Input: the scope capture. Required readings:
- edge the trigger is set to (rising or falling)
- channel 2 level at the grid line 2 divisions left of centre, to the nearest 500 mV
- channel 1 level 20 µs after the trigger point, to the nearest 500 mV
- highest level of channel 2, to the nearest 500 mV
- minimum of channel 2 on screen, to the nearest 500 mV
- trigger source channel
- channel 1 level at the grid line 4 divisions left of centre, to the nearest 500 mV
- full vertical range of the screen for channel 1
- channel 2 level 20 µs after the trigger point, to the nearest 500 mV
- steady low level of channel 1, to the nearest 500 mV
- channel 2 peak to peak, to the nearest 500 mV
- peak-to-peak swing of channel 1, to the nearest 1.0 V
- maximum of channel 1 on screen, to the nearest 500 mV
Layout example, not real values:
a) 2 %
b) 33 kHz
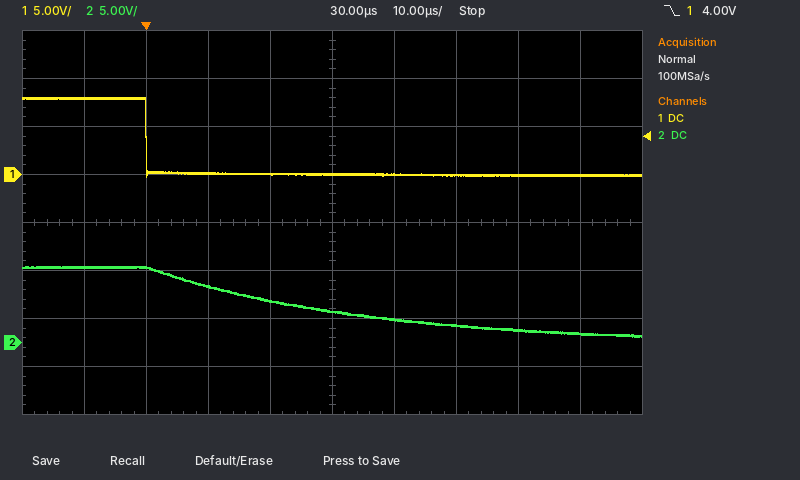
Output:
a) falling
b) 6.0 V
c) 0.0 V
d) 8.0 V
e) 500 mV
f) channel 1
g) 8.0 V
h) 40 V
i) 4.5 V
j) 0.0 V
k) 7.5 V
l) 8.0 V
m) 8.0 V
